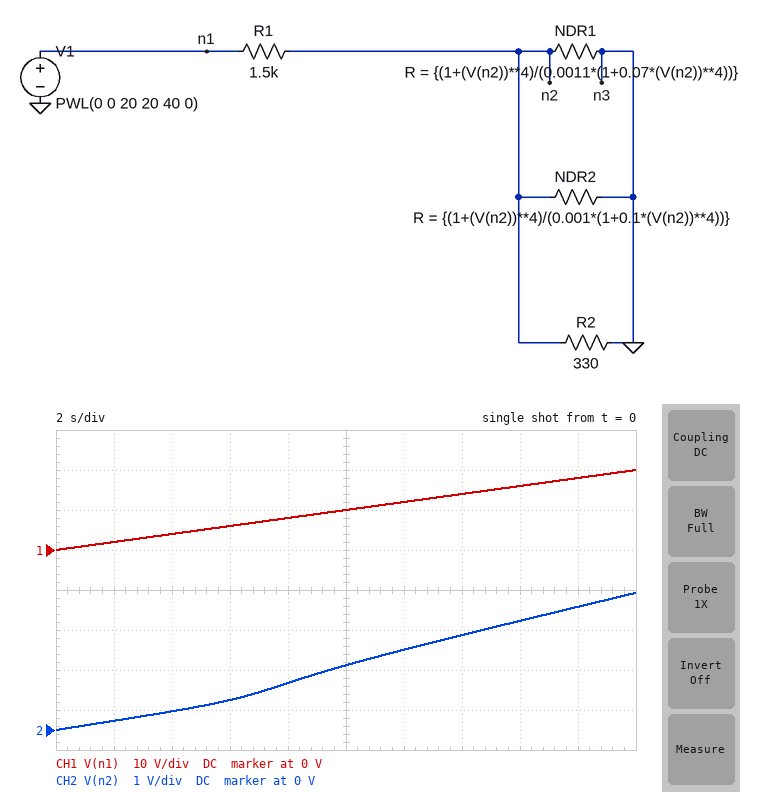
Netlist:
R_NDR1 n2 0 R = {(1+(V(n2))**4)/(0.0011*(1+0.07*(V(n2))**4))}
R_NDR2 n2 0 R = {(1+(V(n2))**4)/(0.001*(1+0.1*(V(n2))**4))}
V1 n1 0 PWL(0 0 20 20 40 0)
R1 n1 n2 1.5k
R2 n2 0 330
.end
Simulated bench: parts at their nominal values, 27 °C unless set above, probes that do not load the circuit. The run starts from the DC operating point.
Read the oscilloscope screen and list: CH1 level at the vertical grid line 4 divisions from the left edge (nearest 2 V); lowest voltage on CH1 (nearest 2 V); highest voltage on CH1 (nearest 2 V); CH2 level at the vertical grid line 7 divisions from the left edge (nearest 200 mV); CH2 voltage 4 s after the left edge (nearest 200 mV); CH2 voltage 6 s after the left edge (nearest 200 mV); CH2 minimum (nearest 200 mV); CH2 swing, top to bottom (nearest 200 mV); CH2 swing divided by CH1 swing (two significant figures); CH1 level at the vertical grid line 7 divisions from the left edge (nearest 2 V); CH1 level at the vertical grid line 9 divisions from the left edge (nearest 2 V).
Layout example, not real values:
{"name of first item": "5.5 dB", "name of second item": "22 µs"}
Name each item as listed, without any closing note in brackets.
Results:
{"CH1 level at the vertical grid line 4 divisions from the left edge": "8 V", "lowest voltage on CH1": "0 V", "highest voltage on CH1": "20 V", "CH2 level at the vertical grid line 7 divisions from the left edge": "2.4 V", "CH2 voltage 4 s after the left edge": "400 mV", "CH2 voltage 6 s after the left edge": "800 mV", "CH2 minimum": "0 V", "CH2 swing, top to bottom": "3.4 V", "CH2 swing divided by CH1 swing": "0.17", "CH1 level at the vertical grid line 7 divisions from the left edge": "14 V", "CH1 level at the vertical grid line 9 divisions from the left edge": "18 V"}
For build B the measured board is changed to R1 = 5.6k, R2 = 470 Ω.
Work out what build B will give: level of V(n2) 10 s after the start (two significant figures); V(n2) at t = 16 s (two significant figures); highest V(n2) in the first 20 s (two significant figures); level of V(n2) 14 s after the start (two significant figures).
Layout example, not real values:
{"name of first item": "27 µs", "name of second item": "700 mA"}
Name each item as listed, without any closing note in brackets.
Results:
{"level of V(n2) 10 s after the start": "410 mV", "V(n2) at t = 16 s": "710 mV", "highest V(n2) in the first 20 s": "1.1 V", "level of V(n2) 14 s after the start": "600 mV"}
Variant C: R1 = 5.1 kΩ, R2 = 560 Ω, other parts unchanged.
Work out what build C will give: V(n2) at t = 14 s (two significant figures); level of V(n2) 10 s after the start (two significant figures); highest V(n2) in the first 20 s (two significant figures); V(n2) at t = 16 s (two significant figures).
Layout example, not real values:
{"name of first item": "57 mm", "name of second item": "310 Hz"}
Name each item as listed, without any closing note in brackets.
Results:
{"V(n2) at t = 14 s": "760 mV", "level of V(n2) 10 s after the start": "490 mV", "highest V(n2) in the first 20 s": "1.6 V", "V(n2) at t = 16 s": "1.0 V"}
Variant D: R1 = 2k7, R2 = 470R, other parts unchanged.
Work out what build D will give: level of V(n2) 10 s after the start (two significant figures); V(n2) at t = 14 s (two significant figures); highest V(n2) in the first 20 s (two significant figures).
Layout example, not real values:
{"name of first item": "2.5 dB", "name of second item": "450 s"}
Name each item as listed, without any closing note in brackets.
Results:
{"level of V(n2) 10 s after the start": "1.0 V", "V(n2) at t = 14 s": "1.8 V", "highest V(n2) in the first 20 s": "2.7 V"}
